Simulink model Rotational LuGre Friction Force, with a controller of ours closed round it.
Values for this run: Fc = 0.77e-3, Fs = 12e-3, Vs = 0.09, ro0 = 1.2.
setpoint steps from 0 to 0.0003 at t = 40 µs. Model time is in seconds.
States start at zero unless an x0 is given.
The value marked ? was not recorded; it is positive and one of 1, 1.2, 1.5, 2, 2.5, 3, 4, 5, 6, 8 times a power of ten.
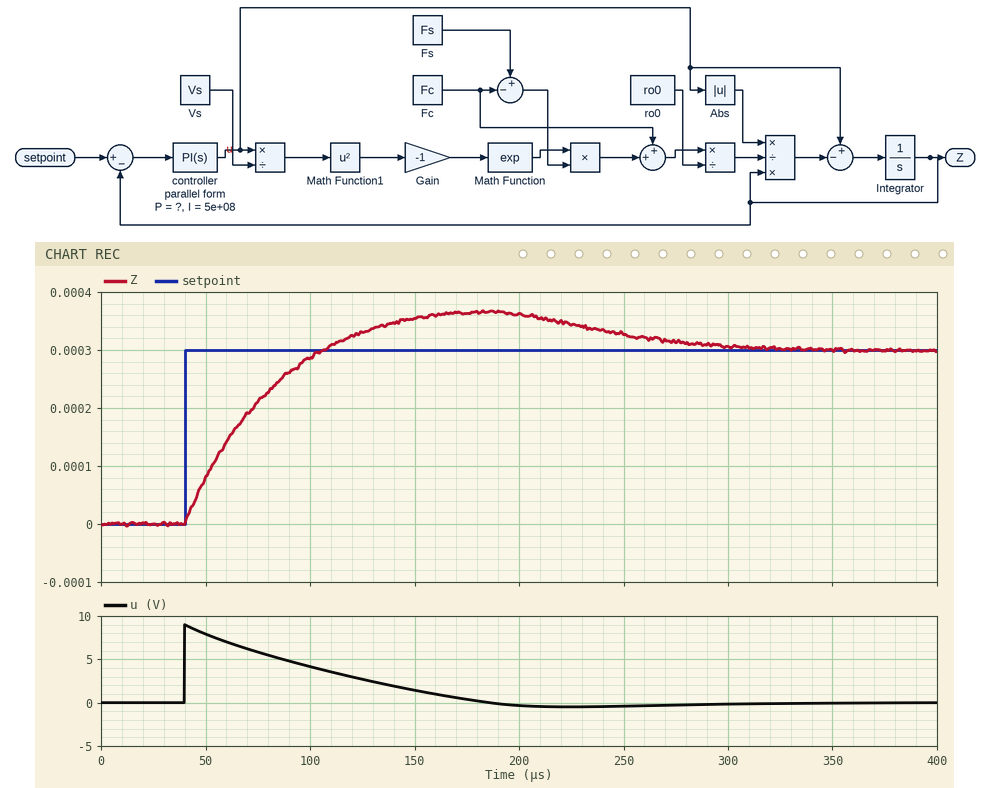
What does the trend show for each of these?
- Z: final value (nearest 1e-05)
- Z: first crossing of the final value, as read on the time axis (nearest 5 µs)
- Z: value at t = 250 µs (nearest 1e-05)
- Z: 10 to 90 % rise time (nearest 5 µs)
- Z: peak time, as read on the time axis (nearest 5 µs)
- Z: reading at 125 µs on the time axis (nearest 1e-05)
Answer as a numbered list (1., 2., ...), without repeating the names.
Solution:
1. 0.00030
2. 105 µs
3. 0.00033
4. 50 µs
5. 185 µs
6. 0.00033
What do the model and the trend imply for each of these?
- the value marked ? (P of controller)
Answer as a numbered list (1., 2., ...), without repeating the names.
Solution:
1. 30000
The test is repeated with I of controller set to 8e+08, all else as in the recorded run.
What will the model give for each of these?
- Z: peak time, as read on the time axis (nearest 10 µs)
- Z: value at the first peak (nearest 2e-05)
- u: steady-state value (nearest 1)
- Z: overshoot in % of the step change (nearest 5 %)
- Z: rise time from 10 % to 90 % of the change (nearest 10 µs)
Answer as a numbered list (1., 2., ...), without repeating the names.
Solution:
1. 160 µs
2. 0.00038
3. 0
4. 25 %
5. 40 µs
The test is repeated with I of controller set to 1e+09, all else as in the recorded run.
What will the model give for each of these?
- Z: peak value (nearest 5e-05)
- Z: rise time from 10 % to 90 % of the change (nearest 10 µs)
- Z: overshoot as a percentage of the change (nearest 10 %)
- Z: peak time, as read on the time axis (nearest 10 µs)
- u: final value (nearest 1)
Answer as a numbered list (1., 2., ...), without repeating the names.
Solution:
1. 0.00040
2. 40 µs
3. 30 %
4. 150 µs
5. 0
